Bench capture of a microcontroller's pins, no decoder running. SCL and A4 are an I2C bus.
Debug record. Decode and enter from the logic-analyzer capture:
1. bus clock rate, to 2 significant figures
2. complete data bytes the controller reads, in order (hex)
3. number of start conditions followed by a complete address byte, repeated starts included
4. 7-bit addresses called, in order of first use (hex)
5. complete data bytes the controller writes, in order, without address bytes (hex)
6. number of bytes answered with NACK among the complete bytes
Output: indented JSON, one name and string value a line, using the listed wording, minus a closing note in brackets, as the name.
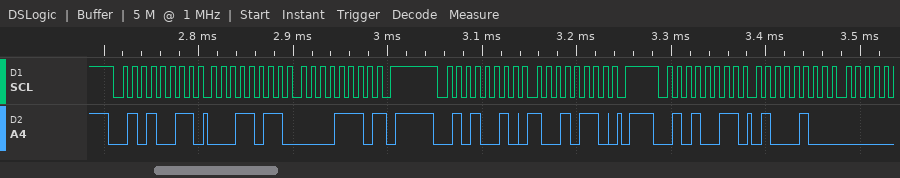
{
  "bus clock rate, to 2 significant figures": "100 kHz",
  "complete data bytes the controller reads, in order": "1B 0E 44",
  "number of start conditions followed by a complete address byte, repeated starts included": "3",
  "7-bit addresses called, in order of first use": "0x29",
  "complete data bytes the controller writes, in order, without address bytes": "96",
  "number of bytes answered with NACK among the complete bytes": "1"
}
